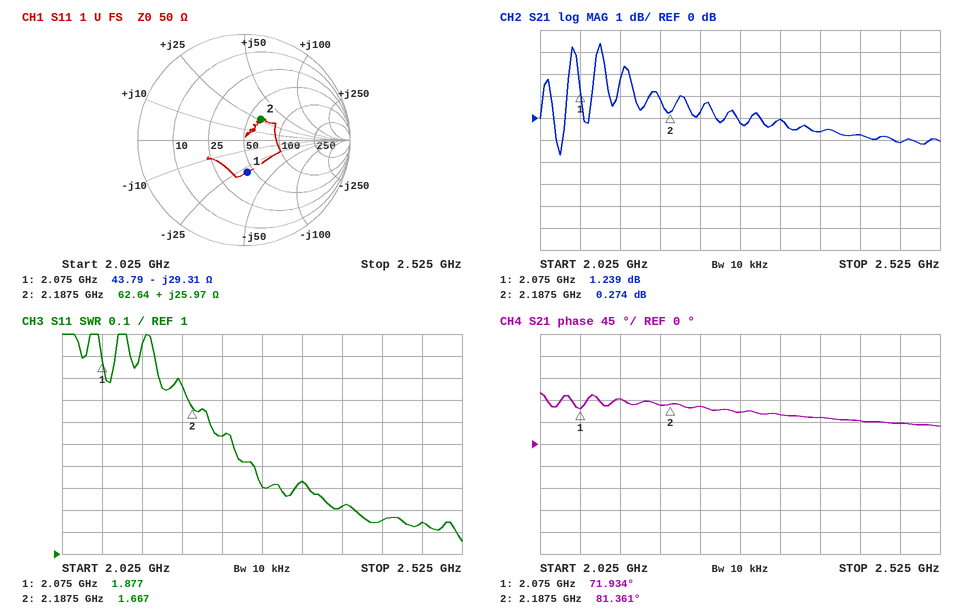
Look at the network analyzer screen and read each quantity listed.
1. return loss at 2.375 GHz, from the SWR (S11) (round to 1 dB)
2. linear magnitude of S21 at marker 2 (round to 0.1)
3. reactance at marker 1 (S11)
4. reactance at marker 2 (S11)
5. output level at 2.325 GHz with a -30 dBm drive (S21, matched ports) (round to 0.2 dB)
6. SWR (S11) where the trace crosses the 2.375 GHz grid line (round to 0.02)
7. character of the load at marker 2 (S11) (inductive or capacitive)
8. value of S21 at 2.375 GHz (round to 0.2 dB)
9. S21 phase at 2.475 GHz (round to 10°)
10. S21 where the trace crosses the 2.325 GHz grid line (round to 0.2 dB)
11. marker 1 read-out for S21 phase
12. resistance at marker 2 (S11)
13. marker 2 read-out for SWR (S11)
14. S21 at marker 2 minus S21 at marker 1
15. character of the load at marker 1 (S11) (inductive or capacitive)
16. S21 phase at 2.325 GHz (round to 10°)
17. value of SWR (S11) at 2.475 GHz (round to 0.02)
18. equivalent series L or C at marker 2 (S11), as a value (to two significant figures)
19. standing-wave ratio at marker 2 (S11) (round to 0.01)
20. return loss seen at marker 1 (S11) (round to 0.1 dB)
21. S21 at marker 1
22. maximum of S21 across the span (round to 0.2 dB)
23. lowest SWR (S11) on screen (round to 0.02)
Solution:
20 dB
1.0
-29.31 Ω
+25.97 Ω
-30.0 dBm
1.22
inductive
-0.6 dB
40°
0.0 dB
71.934°
62.64 Ω
1.667
-0.965 dB
capacitive
60°
1.14
1.9 nH
1.67
10.3 dB
1.239 dB
3.4 dB
1.06
